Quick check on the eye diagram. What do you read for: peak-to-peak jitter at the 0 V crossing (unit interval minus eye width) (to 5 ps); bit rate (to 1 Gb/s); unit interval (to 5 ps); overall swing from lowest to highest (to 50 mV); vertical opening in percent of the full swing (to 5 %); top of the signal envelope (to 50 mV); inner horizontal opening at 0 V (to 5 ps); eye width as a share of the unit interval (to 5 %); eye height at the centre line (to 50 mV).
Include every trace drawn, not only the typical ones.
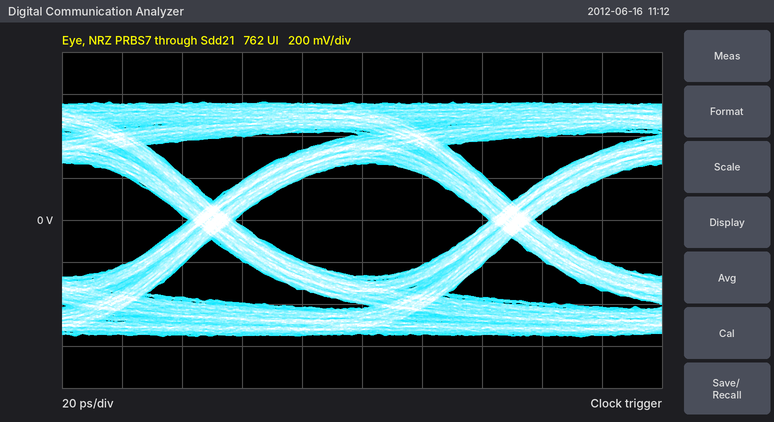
15 ps
10 Gb/s
100 ps
1.10 V
50 %
550 mV
85 ps
85 %
550 mV
